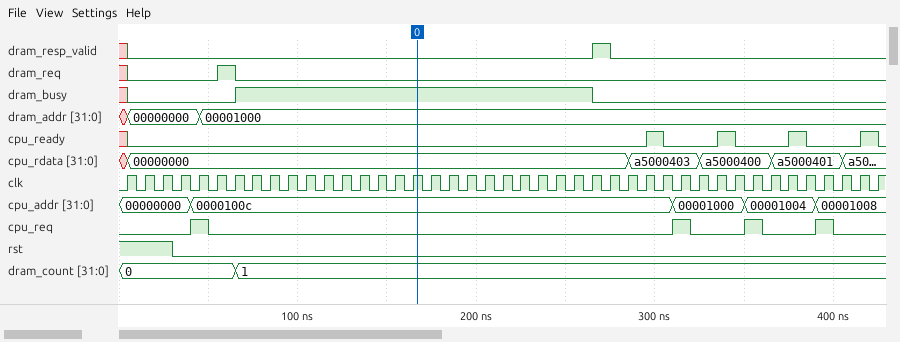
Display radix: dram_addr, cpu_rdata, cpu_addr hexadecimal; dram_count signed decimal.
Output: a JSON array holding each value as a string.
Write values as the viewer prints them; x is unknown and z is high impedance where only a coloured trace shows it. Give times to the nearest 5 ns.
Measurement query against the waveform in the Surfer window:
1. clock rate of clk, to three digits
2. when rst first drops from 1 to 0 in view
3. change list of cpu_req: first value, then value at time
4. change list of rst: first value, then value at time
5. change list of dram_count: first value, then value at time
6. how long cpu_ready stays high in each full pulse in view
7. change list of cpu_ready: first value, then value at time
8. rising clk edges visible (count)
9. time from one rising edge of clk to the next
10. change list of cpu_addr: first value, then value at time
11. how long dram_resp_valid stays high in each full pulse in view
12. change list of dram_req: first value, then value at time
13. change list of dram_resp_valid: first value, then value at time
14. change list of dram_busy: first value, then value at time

["100 MHz", "30 ns", "0, 1 at 40 ns, 0 at 50 ns, 1 at 310 ns, 0 at 320 ns, 1 at 350 ns, 0 at 360 ns, 1 at 390 ns, 0 at 400 ns", "1, 0 at 30 ns", "0, 1 at 65 ns", "10 ns, 10 ns, 10 ns, 10 ns", "x, 0 at 5 ns, 1 at 295 ns, 0 at 305 ns, 1 at 335 ns, 0 at 345 ns, 1 at 375 ns, 0 at 385 ns, 1 at 415 ns, 0 at 425 ns", "43", "10 ns", "00000000, 0000100c at 40 ns, 00001000 at 310 ns, 00001004 at 350 ns, 00001008 at 390 ns", "10 ns", "x, 0 at 5 ns, 1 at 55 ns, 0 at 65 ns", "x, 0 at 5 ns, 1 at 265 ns, 0 at 275 ns", "x, 0 at 5 ns, 1 at 65 ns, 0 at 265 ns"]
